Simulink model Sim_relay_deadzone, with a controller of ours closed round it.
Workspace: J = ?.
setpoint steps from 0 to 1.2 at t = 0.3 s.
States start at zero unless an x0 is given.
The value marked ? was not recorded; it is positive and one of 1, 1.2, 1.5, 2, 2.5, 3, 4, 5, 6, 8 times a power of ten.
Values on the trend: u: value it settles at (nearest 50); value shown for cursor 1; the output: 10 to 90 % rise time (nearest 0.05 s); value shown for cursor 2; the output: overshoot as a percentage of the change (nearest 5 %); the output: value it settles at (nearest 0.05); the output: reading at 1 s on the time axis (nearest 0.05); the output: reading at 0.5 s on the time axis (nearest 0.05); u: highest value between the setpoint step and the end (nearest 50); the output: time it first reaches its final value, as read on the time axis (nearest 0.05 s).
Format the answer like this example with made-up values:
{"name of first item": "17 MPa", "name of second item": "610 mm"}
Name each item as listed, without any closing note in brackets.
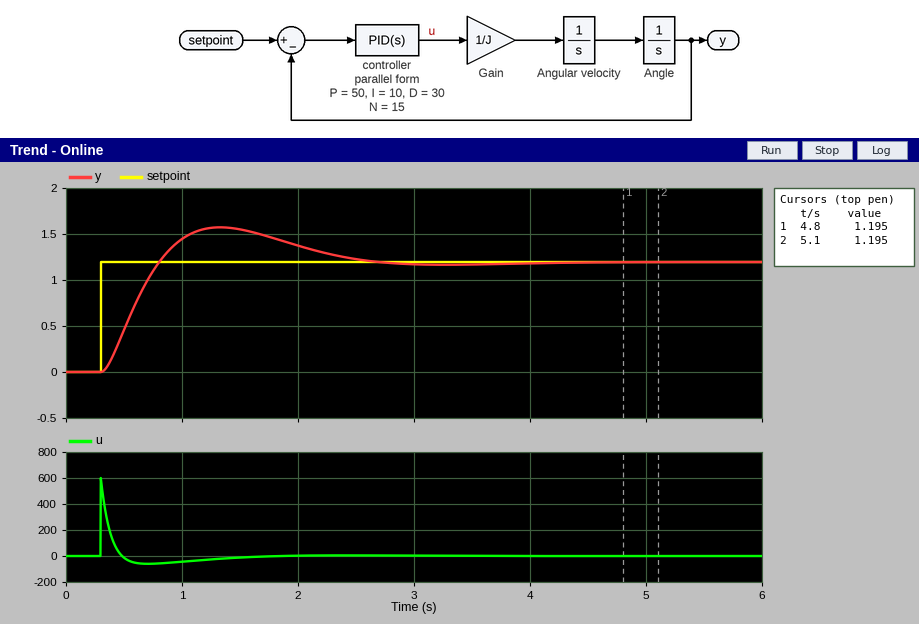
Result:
{"u: value it settles at": "0", "value shown for cursor 1": "1.195", "the output: 10 to 90 % rise time": "0.35 s", "value shown for cursor 2": "1.195", "the output: overshoot as a percentage of the change": "30 %", "the output: value it settles at": "1.20", "the output: reading at 1 s on the time axis": "1.45", "the output: reading at 0.5 s on the time axis": "0.45", "u: highest value between the setpoint step and the end": "600", "the output: time it first reaches its final value, as read on the time axis": "0.80 s"}
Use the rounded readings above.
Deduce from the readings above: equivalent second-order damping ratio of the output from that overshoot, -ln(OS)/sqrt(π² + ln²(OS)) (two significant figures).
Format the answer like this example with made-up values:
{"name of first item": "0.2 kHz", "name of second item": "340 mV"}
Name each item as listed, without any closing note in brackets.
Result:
{"equivalent second-order damping ratio of the output from that overshoot, -ln(OS)/sqrt(π² + ln²(OS))": "0.36"}
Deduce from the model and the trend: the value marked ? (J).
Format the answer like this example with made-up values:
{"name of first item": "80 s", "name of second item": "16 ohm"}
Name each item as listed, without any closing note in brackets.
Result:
{"the value marked ?": "12"}
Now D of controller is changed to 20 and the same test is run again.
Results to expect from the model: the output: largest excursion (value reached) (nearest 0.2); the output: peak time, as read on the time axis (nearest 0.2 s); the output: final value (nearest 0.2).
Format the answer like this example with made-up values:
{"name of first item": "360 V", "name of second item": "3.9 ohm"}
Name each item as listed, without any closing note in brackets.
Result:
{"the output: largest excursion (value reached)": "1.8", "the output: peak time, as read on the time axis": "1.4 s", "the output: final value": "1.2"}
